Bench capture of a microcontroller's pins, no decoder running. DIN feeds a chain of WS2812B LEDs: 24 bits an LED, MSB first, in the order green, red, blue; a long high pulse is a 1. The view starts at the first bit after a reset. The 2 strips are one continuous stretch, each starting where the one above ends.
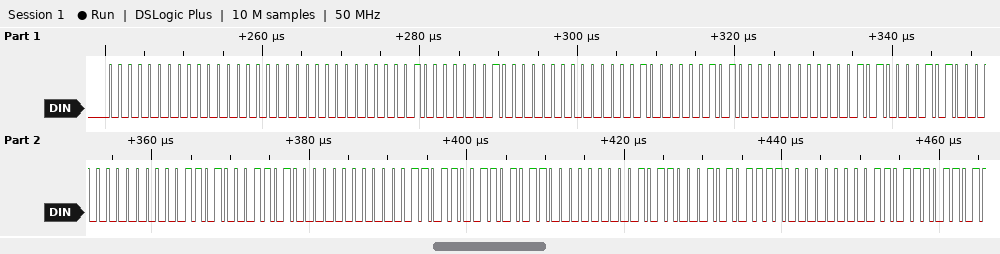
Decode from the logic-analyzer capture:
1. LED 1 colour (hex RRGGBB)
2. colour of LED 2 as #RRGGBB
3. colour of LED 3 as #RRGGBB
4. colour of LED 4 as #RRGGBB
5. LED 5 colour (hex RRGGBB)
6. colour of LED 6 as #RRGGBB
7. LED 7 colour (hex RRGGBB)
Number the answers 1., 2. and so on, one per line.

1. #000000
2. #010100
3. #050200
4. #140A00
5. #341A00
6. #6B3600
7. #AF5800
